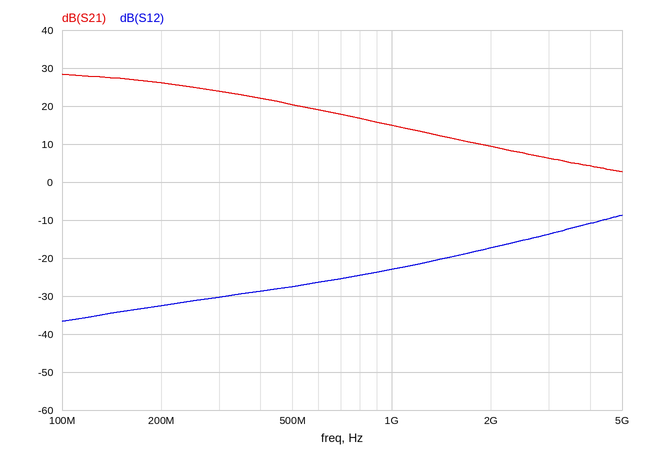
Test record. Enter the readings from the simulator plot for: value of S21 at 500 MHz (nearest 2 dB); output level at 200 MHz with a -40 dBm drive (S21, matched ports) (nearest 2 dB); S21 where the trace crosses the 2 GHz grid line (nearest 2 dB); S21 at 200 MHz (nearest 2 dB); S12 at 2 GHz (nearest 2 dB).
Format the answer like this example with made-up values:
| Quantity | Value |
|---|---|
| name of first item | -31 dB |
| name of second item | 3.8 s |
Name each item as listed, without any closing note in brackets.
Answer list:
| Quantity | Value |
|---|---|
| value of S21 at 500 MHz | 20 dB |
| output level at 200 MHz with a -40 dBm drive (S21, matched ports) | -14 dBm |
| S21 where the trace crosses the 2 GHz grid line | 10 dB |
| S21 at 200 MHz | 26 dB |
| S12 at 2 GHz | -18 dB |
